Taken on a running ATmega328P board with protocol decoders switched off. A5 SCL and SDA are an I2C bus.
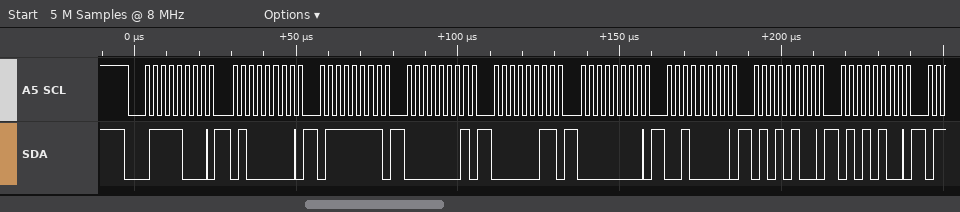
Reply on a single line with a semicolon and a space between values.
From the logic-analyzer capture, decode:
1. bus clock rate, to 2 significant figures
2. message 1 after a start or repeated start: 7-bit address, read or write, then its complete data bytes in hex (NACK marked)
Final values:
400 kHz; 0x3C write: 40 7F 01 03 00 20 54 54
